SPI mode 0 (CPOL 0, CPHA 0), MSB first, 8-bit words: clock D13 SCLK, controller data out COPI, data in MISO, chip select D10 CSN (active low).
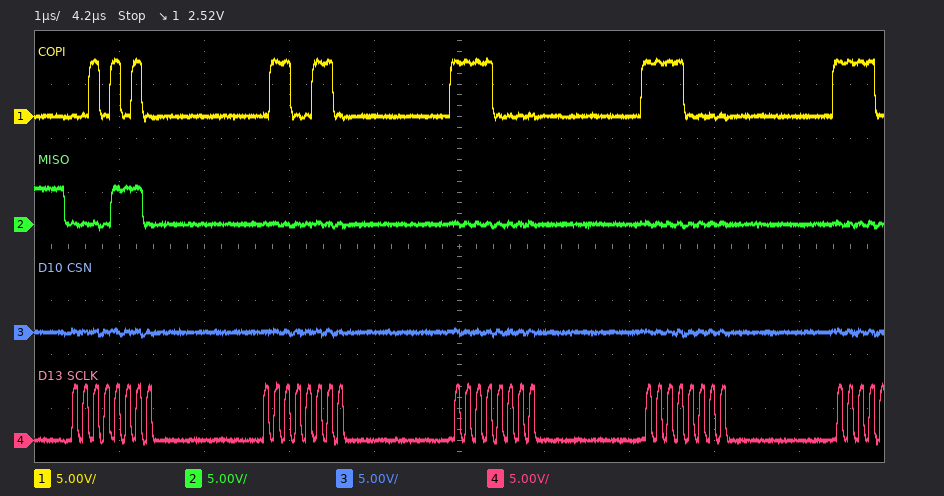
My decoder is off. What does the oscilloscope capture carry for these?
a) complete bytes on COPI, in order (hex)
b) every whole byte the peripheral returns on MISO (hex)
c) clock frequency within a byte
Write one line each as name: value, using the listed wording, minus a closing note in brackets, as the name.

complete bytes on COPI, in order: 2A 66 F0 F0
every whole byte the peripheral returns on MISO: 0E 00 00 00
clock frequency within a byte: 8 MHz
